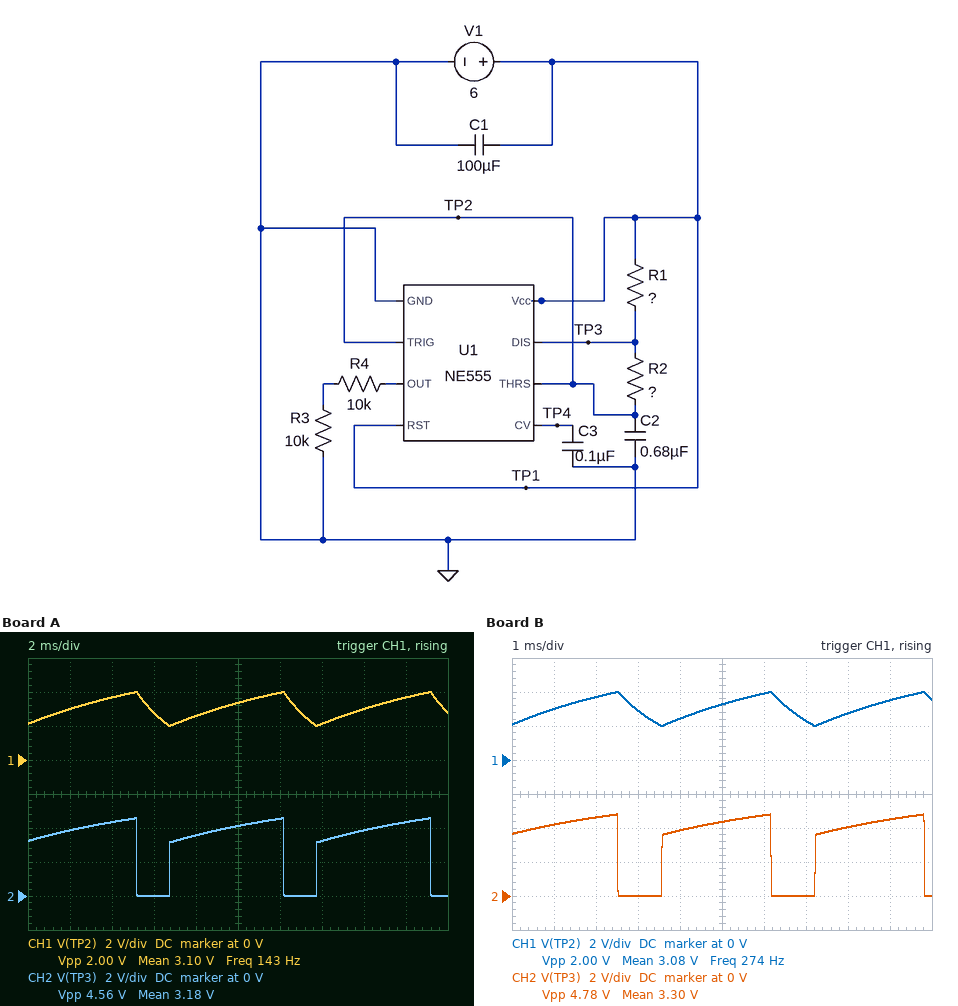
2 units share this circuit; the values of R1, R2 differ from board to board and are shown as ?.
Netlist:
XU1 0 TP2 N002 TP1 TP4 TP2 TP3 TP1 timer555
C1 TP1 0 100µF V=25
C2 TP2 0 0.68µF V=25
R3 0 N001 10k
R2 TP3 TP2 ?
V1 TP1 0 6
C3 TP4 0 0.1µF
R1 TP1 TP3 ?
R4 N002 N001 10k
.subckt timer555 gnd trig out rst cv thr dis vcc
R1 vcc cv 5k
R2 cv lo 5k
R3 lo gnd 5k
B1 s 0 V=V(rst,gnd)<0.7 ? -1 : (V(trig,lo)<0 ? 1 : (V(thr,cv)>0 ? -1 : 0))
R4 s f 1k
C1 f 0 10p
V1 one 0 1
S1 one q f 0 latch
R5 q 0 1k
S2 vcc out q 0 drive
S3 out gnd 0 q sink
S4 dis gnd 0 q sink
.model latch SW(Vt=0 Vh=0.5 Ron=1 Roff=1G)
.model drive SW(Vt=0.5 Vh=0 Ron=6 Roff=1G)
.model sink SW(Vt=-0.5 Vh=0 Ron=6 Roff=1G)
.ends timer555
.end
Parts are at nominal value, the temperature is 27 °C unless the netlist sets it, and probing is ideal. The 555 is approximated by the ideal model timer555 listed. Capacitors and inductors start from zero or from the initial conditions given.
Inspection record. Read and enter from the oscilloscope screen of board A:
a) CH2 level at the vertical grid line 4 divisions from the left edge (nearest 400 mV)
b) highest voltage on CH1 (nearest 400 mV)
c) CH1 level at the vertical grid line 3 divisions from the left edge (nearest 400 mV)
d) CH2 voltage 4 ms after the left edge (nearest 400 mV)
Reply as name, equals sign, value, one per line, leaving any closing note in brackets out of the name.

CH2 level at the vertical grid line 4 divisions from the left edge = 3.6 V
highest voltage on CH1 = 4.0 V
CH1 level at the vertical grid line 3 divisions from the left edge = 2.8 V
CH2 voltage 4 ms after the left edge = 4.4 V
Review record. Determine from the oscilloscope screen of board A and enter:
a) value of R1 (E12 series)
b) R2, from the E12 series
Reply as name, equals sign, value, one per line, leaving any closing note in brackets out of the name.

value of R1 = 8.2 kΩ
R2, from the E12 series = 3.3 kΩ
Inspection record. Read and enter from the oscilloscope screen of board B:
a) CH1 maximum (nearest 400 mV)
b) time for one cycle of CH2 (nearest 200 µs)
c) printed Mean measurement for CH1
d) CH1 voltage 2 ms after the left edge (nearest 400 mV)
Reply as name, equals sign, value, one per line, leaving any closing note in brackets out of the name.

CH1 maximum = 4.0 V
time for one cycle of CH2 = 3.6 ms
printed Mean measurement for CH1 = 3.08 V
CH1 voltage 2 ms after the left edge = 3.6 V
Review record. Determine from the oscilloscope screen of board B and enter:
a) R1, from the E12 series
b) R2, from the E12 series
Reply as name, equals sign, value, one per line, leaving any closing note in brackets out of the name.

R1, from the E12 series = 3.3 kΩ
R2, from the E12 series = 2.2 kΩ
